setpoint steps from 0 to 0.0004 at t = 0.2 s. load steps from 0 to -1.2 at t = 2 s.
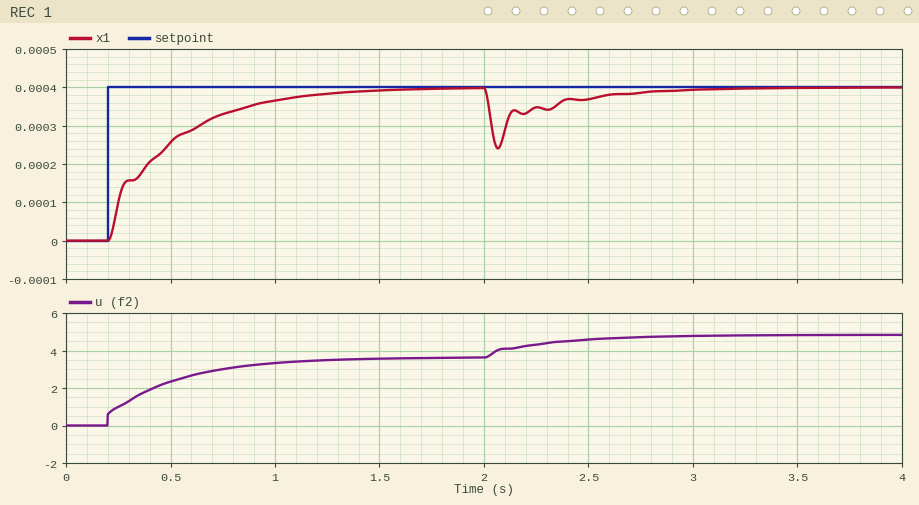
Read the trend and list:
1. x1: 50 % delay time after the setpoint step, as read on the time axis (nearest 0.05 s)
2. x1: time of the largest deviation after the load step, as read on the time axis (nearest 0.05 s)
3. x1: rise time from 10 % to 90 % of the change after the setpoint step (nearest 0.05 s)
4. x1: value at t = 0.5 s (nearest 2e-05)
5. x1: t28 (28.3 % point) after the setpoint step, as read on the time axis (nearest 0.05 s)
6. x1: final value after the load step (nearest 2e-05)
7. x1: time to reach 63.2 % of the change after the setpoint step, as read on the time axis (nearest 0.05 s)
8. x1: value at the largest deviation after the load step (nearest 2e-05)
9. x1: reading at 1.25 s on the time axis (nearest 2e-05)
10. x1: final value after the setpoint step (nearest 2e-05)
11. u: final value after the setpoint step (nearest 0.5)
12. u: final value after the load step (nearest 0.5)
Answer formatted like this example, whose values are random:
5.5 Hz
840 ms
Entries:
0.40 s
2.05 s
0.70 s
0.00026
0.25 s
0.00040
0.50 s
0.00024
0.00038
0.00040
3.5
5.0
